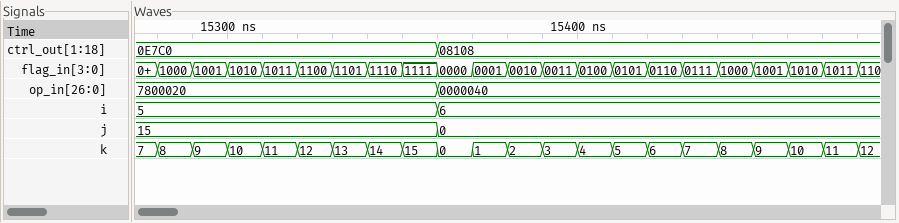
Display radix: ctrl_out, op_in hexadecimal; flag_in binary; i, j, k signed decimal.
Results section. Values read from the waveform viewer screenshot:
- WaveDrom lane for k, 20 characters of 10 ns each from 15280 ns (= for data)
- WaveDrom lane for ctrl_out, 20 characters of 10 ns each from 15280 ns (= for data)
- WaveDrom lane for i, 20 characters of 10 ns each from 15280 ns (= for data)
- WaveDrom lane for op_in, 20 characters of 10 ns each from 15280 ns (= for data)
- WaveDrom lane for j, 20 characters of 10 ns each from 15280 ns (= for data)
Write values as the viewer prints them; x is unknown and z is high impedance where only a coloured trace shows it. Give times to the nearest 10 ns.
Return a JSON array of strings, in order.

["{name: 'k', wave: '====================', data: '8 9 10 11 12 13 14 15 0 1 2 3 4 5 6 7 8 9 10 11'}", "{name: 'ctrl_out', wave: '=.......=...........', data: '0E7C0 08108'}", "{name: 'i', wave: '=.......=...........', data: '5 6'}", "{name: 'op_in', wave: '=.......=...........', data: '7800020 0000040'}", "{name: 'j', wave: '=.......=...........', data: '15 0'}"]
